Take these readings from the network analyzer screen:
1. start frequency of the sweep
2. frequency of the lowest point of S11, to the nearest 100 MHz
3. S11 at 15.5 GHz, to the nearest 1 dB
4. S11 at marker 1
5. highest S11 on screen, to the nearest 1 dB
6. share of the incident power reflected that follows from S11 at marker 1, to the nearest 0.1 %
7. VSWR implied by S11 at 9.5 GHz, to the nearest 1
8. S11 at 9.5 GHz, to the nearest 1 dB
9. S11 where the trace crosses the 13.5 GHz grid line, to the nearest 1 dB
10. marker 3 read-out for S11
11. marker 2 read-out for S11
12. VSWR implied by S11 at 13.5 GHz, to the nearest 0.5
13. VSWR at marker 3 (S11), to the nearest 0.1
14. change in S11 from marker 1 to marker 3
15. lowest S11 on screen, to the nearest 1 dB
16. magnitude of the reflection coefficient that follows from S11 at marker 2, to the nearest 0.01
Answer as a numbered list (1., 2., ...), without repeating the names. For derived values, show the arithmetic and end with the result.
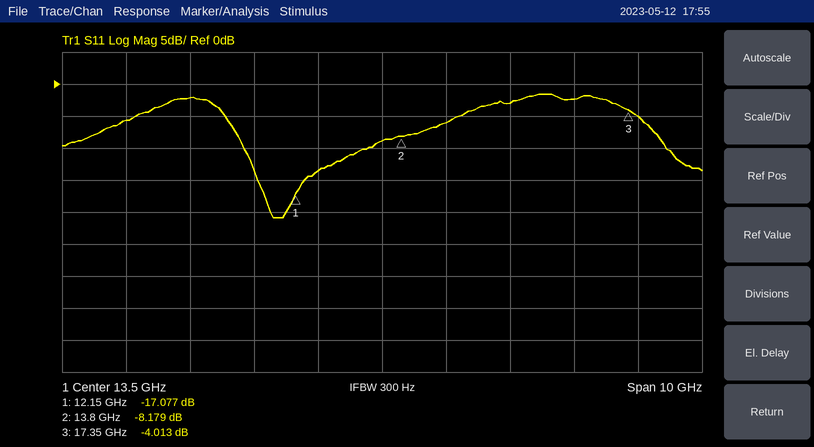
1. 8.5 GHz
2. 11.8 GHz
3. -3 dB
4. -17.077 dB
5. -2 dB
6. 10^(-17.077/10) ≈ 2.0 %
7. |Γ| = 10^(-6/20) = 0.5012; VSWR = (1 + 0.5012)/(1 − 0.5012) ≈ 3
8. -6 dB
9. -9 dB
10. -4.013 dB
11. -8.179 dB
12. |Γ| = 10^(-9/20) = 0.3548; VSWR = (1 + 0.3548)/(1 − 0.3548) ≈ 2.10, so 2.0 to the nearest 0.5
13. (1 + 0.6300)/(1 − 0.6300) ≈ 4.4
14. -4.013 − (-17.077) = 13.064 dB
15. -21 dB
16. 10^(-8.179/20) ≈ 0.39
